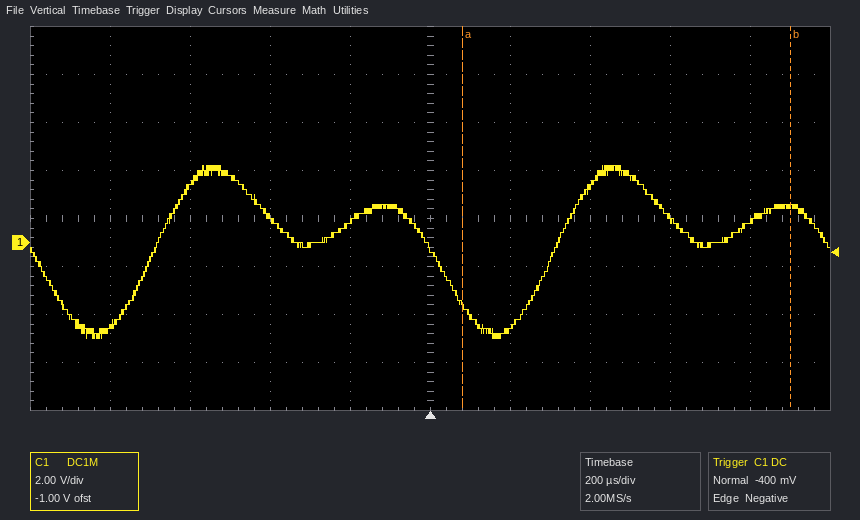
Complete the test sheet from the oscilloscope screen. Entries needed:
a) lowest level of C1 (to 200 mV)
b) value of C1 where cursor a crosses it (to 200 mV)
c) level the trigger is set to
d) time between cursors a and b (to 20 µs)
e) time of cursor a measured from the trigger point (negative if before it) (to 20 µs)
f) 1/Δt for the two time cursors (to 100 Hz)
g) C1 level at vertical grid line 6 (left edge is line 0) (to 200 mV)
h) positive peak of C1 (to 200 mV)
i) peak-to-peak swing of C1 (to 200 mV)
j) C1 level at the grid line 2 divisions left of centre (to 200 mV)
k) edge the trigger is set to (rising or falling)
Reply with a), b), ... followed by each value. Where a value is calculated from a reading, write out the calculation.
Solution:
a) -4.0 V
b) -2.6 V
c) -400 mV
d) 820 µs
e) +80 µs
f) 1 / 820 µs ≈ 1.2 kHz
g) -3.6 V
h) 3.2 V
i) 3.2 V − (-4.0 V) = 7.2 V
j) 1.0 V
k) falling
